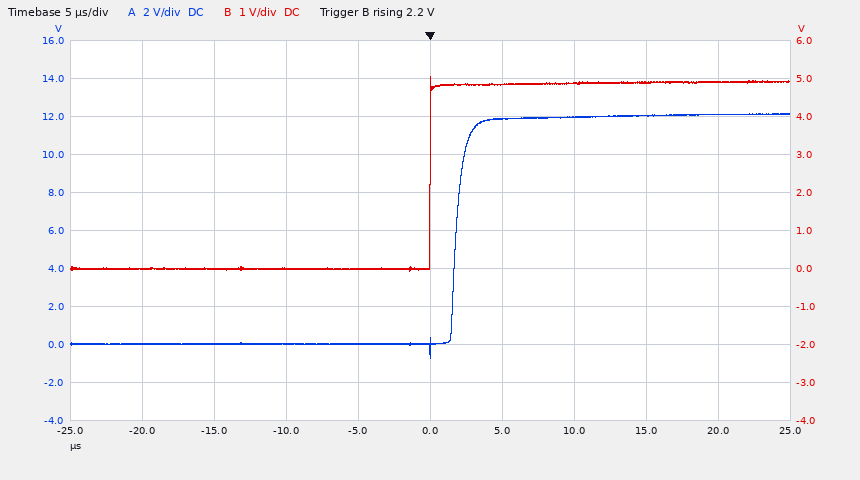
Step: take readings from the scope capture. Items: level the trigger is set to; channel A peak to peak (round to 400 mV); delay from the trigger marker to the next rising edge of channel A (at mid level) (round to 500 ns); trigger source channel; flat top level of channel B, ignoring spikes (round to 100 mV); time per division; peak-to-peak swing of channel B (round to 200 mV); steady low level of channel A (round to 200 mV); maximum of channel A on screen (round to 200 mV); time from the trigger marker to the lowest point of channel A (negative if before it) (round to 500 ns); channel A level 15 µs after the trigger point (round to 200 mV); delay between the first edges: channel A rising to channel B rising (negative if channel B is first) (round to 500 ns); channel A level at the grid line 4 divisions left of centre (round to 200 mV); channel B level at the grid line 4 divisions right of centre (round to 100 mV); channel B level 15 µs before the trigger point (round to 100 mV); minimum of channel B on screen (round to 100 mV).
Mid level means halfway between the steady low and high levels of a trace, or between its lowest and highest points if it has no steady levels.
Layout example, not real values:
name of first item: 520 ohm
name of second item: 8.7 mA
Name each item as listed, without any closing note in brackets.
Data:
level the trigger is set to: 2.2 V
channel A peak to peak: 12.8 V
delay from the trigger marker to the next rising edge of channel A (at mid level): 2.0 µs
trigger source channel: channel B
flat top level of channel B, ignoring spikes: 4.9 V
time per division: 5 µs
peak-to-peak swing of channel B: 5.2 V
steady low level of channel A: 0.0 V
maximum of channel A on screen: 12.2 V
time from the trigger marker to the lowest point of channel A (negative if before it): 0.0 µs
channel A level 15 µs after the trigger point: 12.0 V
delay between the first edges: channel A rising to channel B rising (negative if channel B is first): -2.0 µs
channel A level at the grid line 4 divisions left of centre: 0.0 V
channel B level at the grid line 4 divisions right of centre: 4.9 V
channel B level 15 µs before the trigger point: 0.0 V
minimum of channel B on screen: -100 mV
